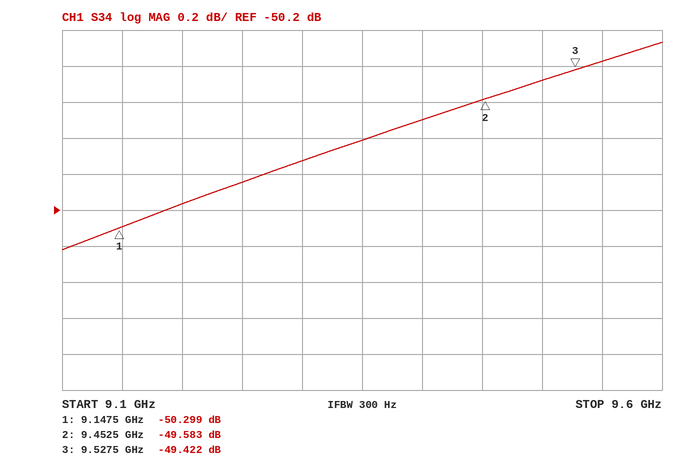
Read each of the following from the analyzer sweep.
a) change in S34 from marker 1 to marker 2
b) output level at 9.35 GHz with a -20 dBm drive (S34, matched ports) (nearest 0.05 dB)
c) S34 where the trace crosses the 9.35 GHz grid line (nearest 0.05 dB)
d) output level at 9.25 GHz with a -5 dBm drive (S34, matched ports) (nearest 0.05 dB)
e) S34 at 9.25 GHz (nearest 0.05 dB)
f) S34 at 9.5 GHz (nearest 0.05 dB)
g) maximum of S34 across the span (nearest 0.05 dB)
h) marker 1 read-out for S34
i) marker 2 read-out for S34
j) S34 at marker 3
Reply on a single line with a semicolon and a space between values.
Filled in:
0.716 dB; -69.80 dBm; -49.80 dB; -55.05 dBm; -50.05 dB; -49.50 dB; -49.25 dB; -50.299 dB; -49.583 dB; -49.422 dB
